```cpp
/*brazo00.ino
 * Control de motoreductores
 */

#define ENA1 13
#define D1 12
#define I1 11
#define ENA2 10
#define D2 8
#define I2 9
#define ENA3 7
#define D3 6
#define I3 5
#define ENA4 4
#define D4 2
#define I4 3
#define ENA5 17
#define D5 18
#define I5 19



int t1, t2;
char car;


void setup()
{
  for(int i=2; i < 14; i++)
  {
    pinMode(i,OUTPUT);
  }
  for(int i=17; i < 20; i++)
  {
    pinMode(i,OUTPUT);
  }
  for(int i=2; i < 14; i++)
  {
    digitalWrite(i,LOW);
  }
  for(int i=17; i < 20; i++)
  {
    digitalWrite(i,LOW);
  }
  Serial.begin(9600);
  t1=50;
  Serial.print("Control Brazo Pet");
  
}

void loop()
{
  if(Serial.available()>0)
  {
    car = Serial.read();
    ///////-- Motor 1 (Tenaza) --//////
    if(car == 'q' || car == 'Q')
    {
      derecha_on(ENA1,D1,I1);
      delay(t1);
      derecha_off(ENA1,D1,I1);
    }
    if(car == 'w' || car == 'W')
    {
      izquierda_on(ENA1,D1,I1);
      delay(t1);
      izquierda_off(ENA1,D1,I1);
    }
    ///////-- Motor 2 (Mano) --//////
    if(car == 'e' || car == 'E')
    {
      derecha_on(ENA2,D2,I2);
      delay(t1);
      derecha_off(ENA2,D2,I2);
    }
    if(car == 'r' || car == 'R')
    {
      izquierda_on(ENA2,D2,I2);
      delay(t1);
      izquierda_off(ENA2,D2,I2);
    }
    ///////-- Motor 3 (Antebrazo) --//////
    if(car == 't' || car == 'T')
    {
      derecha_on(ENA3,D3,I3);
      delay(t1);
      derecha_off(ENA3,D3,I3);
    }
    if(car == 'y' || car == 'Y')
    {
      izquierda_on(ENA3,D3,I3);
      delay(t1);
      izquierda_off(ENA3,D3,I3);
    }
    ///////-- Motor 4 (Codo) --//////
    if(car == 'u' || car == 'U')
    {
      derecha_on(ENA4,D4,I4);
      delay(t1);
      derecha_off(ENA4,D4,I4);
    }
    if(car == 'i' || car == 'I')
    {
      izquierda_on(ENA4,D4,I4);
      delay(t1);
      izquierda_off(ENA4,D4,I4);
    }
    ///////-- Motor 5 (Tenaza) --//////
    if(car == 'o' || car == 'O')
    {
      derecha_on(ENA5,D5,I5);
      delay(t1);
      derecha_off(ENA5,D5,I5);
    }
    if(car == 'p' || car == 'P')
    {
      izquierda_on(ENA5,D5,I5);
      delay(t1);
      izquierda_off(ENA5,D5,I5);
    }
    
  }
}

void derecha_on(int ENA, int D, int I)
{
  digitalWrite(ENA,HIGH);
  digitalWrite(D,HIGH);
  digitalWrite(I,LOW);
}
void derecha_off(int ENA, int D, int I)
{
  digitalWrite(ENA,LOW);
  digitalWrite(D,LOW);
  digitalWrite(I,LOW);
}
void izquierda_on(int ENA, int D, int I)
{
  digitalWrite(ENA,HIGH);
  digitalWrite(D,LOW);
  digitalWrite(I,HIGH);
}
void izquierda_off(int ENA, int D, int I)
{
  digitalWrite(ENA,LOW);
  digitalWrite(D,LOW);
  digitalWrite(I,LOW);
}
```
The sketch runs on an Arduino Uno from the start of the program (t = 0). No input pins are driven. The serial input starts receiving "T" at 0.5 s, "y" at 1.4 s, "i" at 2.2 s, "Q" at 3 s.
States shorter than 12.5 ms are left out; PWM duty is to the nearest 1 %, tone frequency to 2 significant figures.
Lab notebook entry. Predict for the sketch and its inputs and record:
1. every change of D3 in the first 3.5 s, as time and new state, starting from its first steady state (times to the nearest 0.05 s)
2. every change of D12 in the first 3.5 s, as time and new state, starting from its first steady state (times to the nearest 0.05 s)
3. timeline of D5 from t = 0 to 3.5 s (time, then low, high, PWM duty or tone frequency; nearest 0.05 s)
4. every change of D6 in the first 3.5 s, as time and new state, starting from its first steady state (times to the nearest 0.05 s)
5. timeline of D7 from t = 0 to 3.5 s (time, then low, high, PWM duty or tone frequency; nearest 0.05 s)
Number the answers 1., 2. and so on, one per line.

1. 0 s low; 2.2 s high; 2.25 s low
2. 0 s low; 3 s high; 3.05 s low
3. 0 s low; 1.4 s high; 1.45 s low
4. 0 s low; 0.5 s high; 0.55 s low
5. 0 s low; 0.5 s high; 0.55 s low; 1.4 s high; 1.45 s low
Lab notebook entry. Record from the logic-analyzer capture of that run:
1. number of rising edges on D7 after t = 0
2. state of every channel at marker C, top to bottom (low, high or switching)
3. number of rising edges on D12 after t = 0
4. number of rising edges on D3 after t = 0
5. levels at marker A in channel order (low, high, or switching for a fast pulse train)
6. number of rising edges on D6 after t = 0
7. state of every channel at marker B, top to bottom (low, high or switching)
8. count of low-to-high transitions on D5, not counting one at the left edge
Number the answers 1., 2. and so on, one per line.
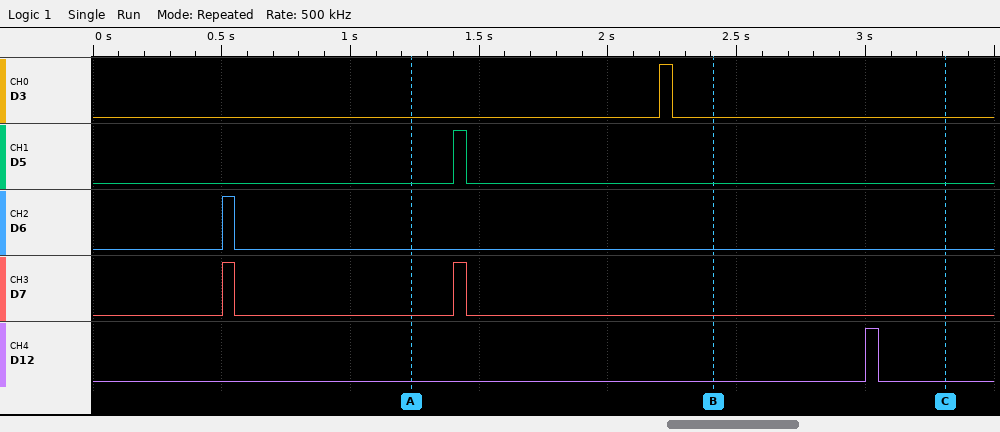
1. 2
2. D3 low, D5 low, D6 low, D7 low, D12 low
3. 1
4. 1
5. D3 low, D5 low, D6 low, D7 low, D12 low
6. 1
7. D3 low, D5 low, D6 low, D7 low, D12 low
8. 1
